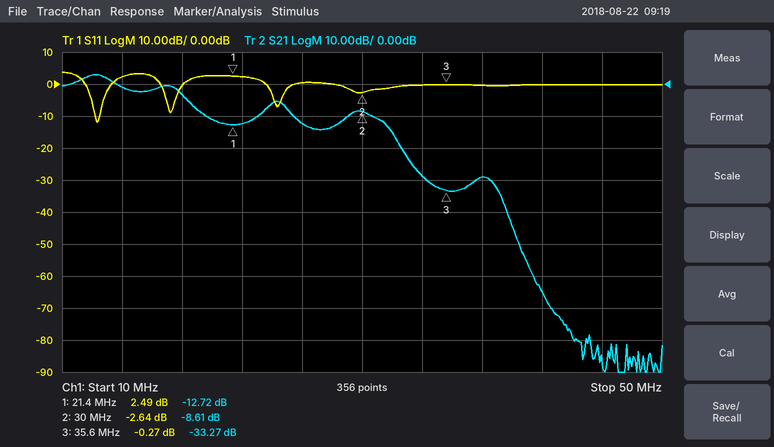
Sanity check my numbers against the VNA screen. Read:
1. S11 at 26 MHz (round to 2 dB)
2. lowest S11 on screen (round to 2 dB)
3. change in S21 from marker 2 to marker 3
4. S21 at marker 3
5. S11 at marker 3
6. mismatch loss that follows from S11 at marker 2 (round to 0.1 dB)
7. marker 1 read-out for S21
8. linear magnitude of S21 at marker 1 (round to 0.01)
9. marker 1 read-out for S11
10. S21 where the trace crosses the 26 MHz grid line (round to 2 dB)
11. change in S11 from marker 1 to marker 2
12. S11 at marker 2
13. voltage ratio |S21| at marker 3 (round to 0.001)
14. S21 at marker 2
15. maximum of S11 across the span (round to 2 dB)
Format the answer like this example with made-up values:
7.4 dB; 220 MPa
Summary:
0 dB; -12 dB; -24.66 dB; -33.27 dB; -0.27 dB; 3.4 dB; -12.72 dB; 0.23; 2.49 dB; -12 dB; -5.13 dB; -2.64 dB; 0.022; -8.61 dB; 4 dB
